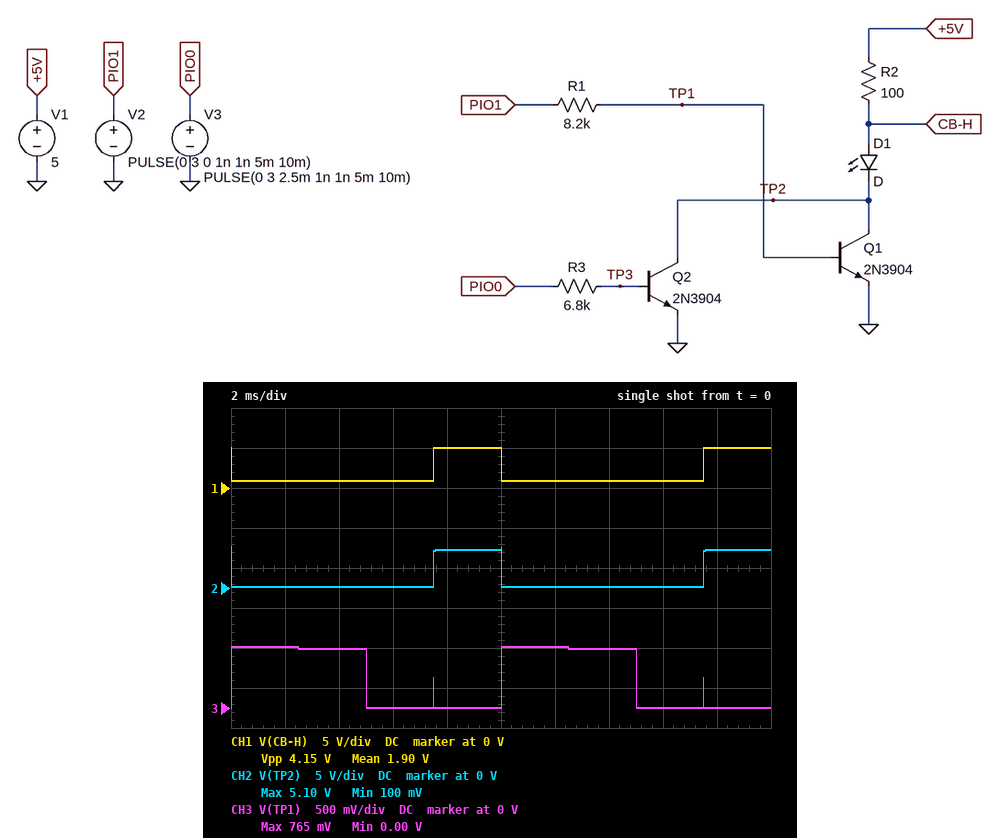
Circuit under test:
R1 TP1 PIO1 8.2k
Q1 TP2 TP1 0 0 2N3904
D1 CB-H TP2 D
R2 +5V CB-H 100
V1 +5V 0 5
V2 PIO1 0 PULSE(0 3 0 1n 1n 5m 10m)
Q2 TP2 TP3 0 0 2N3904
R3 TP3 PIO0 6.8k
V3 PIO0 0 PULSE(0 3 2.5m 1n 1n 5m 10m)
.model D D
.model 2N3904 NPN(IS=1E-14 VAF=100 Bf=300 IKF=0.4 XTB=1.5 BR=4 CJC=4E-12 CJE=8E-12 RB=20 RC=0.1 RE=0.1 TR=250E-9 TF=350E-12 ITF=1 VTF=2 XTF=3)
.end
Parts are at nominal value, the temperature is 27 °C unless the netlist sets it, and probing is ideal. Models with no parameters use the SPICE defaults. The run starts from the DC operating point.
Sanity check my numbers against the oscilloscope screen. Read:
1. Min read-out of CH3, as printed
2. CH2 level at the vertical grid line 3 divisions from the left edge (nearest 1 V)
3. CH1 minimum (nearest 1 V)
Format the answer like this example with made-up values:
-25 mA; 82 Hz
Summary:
0.00 V; 0 V; 1 V
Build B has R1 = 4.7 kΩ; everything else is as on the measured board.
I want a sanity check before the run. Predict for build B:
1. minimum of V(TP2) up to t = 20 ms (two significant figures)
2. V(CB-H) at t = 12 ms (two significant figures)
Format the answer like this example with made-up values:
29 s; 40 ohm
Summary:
79 mV; 850 mV
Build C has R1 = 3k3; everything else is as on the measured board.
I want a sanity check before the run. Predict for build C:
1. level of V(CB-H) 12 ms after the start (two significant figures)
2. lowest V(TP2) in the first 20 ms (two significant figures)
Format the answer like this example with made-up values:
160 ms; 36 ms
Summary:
840 mV; 73 mV
